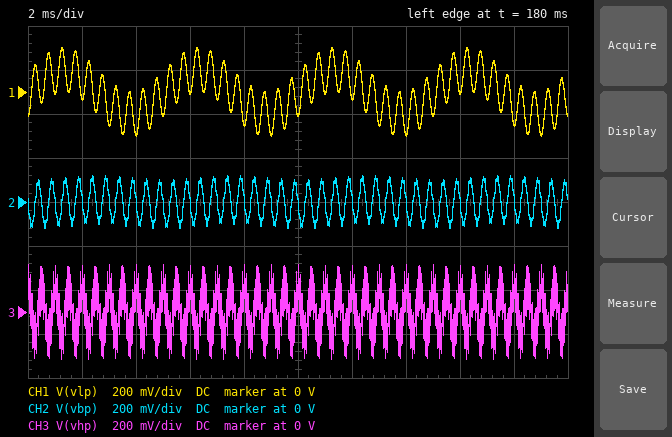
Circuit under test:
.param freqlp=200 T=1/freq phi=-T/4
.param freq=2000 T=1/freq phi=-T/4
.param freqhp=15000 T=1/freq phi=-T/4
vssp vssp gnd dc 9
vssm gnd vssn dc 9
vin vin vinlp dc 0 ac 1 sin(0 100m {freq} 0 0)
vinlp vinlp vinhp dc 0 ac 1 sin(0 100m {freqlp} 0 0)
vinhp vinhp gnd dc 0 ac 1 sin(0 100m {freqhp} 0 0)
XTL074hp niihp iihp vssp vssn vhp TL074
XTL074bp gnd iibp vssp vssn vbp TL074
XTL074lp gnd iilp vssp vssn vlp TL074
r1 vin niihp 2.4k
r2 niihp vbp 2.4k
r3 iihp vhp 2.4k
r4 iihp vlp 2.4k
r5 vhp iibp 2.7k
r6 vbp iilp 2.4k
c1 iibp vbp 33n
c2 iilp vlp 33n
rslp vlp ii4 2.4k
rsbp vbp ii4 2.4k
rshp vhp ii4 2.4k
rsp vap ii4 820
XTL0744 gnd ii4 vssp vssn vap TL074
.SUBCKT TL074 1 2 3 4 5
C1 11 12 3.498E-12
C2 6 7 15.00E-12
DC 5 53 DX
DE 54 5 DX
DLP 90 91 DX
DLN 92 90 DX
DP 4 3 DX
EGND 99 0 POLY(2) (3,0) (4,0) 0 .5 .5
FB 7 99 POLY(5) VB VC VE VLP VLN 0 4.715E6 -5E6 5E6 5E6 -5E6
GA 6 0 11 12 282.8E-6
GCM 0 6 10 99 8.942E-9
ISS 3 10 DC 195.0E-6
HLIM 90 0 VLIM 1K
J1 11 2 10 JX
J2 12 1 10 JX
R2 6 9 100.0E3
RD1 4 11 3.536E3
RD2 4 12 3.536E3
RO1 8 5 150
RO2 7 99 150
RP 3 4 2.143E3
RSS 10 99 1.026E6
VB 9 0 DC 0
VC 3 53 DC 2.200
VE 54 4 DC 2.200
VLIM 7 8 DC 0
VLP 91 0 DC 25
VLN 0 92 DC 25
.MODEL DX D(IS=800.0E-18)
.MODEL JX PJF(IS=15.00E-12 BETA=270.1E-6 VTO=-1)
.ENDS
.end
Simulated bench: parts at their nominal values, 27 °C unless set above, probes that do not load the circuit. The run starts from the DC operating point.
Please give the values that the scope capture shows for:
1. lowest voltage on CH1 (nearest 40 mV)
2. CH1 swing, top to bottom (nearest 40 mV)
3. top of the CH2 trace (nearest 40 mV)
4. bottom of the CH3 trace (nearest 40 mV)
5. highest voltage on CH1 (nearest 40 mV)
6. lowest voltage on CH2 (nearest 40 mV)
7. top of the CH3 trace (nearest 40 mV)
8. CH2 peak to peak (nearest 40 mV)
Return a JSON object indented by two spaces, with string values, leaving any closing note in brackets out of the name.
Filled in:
{
  "lowest voltage on CH1": "-200 mV",
  "CH1 swing, top to bottom": "400 mV",
  "top of the CH2 trace": "120 mV",
  "bottom of the CH3 trace": "-200 mV",
  "highest voltage on CH1": "200 mV",
  "lowest voltage on CH2": "-120 mV",
  "top of the CH3 trace": "200 mV",
  "CH2 peak to peak": "240 mV"
}
